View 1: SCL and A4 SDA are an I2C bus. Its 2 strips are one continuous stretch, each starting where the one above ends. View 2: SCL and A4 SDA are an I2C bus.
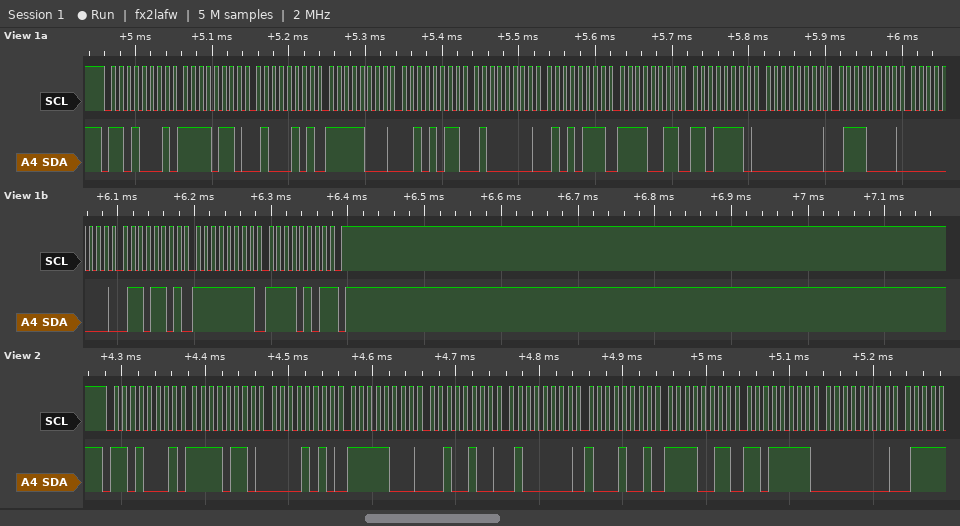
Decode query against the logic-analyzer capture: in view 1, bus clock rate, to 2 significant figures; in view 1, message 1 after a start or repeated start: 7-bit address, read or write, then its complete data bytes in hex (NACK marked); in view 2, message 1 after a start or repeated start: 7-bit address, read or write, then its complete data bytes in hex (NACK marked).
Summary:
100 kHz
0x68 read: F6 45 F8 2B 40 57 F3 DE 00 70 00 6D FF F5 NACK
0x68 read: F6 0A F8 24 40 89 F3 DF 00
